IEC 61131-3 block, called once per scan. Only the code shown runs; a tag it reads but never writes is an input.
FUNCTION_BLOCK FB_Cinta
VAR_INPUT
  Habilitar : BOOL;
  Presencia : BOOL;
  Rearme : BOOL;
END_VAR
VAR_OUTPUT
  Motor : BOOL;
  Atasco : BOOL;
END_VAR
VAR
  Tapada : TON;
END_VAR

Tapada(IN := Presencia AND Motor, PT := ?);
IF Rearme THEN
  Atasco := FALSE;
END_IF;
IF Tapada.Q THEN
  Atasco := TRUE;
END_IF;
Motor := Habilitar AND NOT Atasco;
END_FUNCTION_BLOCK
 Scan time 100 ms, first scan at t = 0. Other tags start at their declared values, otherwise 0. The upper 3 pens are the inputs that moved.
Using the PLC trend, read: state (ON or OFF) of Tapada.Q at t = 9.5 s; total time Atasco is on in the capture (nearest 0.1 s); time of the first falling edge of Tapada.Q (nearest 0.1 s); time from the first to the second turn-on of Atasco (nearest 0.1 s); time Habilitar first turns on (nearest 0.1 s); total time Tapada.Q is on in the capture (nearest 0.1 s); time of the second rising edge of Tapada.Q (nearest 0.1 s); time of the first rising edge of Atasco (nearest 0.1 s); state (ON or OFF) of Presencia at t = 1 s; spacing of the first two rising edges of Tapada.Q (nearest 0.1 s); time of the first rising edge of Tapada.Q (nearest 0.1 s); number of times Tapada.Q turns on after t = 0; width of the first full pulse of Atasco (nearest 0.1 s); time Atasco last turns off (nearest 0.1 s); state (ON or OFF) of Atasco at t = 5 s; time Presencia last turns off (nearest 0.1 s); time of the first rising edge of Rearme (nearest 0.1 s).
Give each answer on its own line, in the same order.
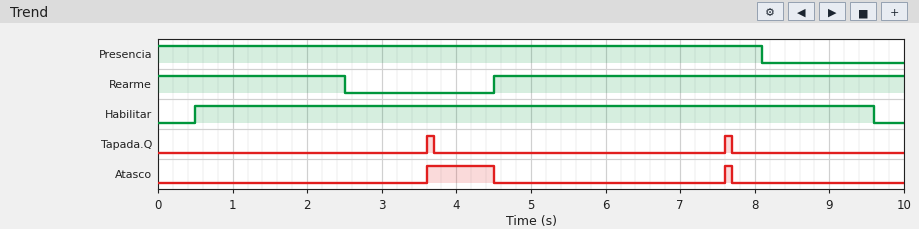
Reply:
OFF
1.0 s
3.7 s
4.0 s
0.5 s
0.2 s
7.6 s
3.6 s
ON
4.0 s
3.6 s
2
0.9 s
7.7 s
OFF
8.1 s
4.5 s
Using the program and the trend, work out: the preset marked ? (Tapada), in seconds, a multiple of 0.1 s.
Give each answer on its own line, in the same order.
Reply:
3.0 s
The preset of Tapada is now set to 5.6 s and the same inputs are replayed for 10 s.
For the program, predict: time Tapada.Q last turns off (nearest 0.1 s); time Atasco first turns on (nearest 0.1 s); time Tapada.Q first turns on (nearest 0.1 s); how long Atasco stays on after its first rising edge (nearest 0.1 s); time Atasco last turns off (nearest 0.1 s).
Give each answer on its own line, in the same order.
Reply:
6.3 s
6.2 s
6.2 s
0.1 s
6.3 s
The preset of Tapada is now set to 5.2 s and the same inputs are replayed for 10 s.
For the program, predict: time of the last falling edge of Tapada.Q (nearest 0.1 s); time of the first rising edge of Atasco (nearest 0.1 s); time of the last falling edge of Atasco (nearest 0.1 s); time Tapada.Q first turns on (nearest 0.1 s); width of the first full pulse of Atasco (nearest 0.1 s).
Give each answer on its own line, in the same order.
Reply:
5.9 s
5.8 s
5.9 s
5.8 s
0.1 s
